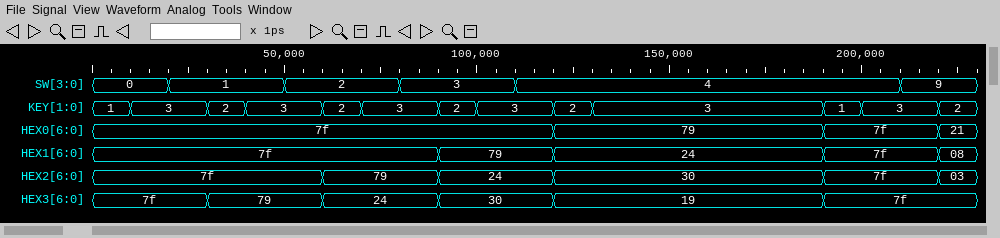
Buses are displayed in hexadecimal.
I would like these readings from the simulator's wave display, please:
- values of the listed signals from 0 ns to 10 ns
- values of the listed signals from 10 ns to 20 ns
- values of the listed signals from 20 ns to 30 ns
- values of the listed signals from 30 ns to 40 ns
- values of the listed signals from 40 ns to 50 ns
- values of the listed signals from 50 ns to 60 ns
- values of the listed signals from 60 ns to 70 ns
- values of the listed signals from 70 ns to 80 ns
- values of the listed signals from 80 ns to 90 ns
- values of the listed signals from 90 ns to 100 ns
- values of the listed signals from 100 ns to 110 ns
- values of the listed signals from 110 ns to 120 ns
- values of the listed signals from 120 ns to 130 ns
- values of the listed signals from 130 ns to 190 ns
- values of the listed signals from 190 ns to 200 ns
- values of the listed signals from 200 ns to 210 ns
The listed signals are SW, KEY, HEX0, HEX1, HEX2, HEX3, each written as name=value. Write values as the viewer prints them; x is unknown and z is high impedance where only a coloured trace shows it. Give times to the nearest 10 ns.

SW=0, KEY=1, HEX0=7f, HEX1=7f, HEX2=7f, HEX3=7f
SW=0, KEY=3, HEX0=7f, HEX1=7f, HEX2=7f, HEX3=7f
SW=1, KEY=3, HEX0=7f, HEX1=7f, HEX2=7f, HEX3=7f
SW=1, KEY=2, HEX0=7f, HEX1=7f, HEX2=7f, HEX3=79
SW=1, KEY=3, HEX0=7f, HEX1=7f, HEX2=7f, HEX3=79
SW=2, KEY=3, HEX0=7f, HEX1=7f, HEX2=7f, HEX3=79
SW=2, KEY=2, HEX0=7f, HEX1=7f, HEX2=79, HEX3=24
SW=2, KEY=3, HEX0=7f, HEX1=7f, HEX2=79, HEX3=24
SW=3, KEY=3, HEX0=7f, HEX1=7f, HEX2=79, HEX3=24
SW=3, KEY=2, HEX0=7f, HEX1=79, HEX2=24, HEX3=30
SW=3, KEY=3, HEX0=7f, HEX1=79, HEX2=24, HEX3=30
SW=4, KEY=3, HEX0=7f, HEX1=79, HEX2=24, HEX3=30
SW=4, KEY=2, HEX0=79, HEX1=24, HEX2=30, HEX3=19
SW=4, KEY=3, HEX0=79, HEX1=24, HEX2=30, HEX3=19
SW=4, KEY=1, HEX0=7f, HEX1=7f, HEX2=7f, HEX3=7f
SW=4, KEY=3, HEX0=7f, HEX1=7f, HEX2=7f, HEX3=7f
